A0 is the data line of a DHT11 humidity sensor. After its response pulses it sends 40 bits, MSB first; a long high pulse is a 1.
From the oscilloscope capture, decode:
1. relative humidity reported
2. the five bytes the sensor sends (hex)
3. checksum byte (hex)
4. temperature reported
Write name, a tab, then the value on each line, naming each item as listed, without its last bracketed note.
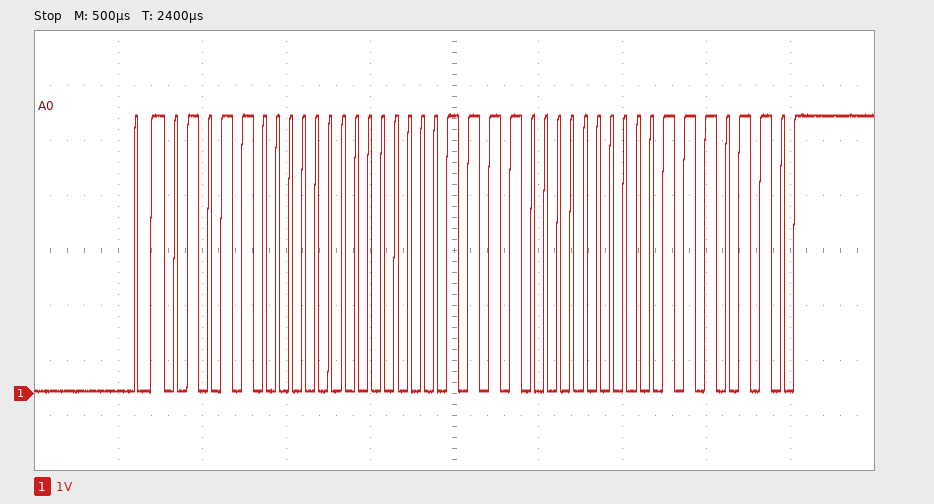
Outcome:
relative humidity reported	88 %
the five bytes the sensor sends	58 00 1E 00 76
checksum byte	0x76
temperature reported	30.0 °C
